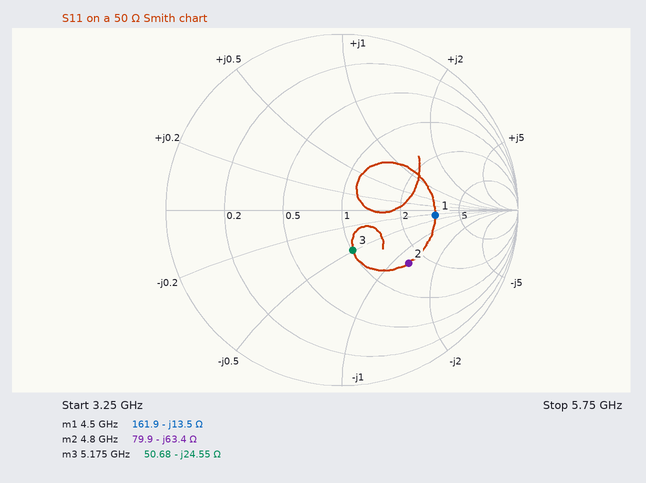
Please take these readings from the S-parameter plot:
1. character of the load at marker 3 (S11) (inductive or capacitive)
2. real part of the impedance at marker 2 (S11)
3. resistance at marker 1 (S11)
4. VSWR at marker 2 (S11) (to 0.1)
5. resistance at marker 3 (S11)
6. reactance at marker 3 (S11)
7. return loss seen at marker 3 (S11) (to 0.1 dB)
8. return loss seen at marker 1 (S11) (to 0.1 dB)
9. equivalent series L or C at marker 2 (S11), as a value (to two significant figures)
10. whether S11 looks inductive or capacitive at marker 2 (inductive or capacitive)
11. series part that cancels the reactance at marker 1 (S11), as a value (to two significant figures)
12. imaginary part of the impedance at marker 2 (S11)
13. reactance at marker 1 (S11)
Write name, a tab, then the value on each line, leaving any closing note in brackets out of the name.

character of the load at marker 3 (S11)	capacitive
real part of the impedance at marker 2	79.9 Ω
resistance at marker 1	161.9 Ω
VSWR at marker 2 (S11)	2.9
resistance at marker 3	50.68 Ω
reactance at marker 3	-24.55 Ω
return loss seen at marker 3 (S11)	12.5 dB
return loss seen at marker 1 (S11)	5.5 dB
equivalent series L or C at marker 2 (S11), as a value	520 fF
whether S11 looks inductive or capacitive at marker 2	capacitive
series part that cancels the reactance at marker 1 (S11), as a value	480 pH
imaginary part of the impedance at marker 2	-63.4 Ω
reactance at marker 1	-13.5 Ω
